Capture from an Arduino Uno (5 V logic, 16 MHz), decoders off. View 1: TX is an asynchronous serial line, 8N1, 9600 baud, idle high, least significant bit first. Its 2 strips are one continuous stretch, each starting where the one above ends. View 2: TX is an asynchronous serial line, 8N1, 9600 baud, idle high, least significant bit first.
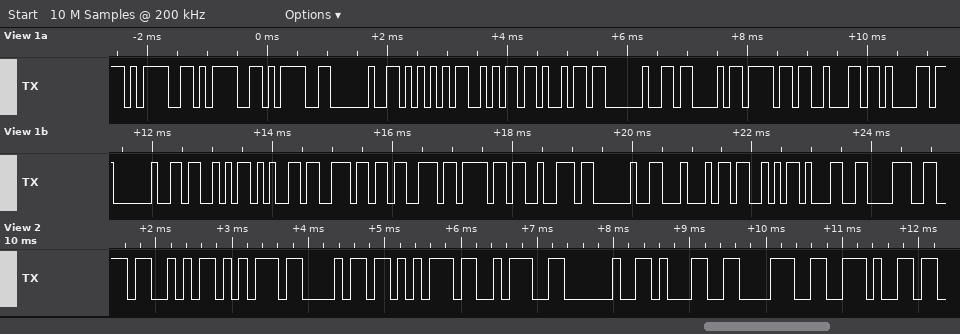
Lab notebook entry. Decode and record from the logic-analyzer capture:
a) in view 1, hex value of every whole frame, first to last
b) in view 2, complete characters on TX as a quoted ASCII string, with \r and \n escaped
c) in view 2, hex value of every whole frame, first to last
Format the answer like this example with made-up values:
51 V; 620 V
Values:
3D 3D 3D 20 55 6A 69 20 43 6F 62 61 20 53 65 6E 73 6F 72 20 44 53 31 38; "Suhu: 18."; 53 75 68 75 3A 20 31 38 2E
